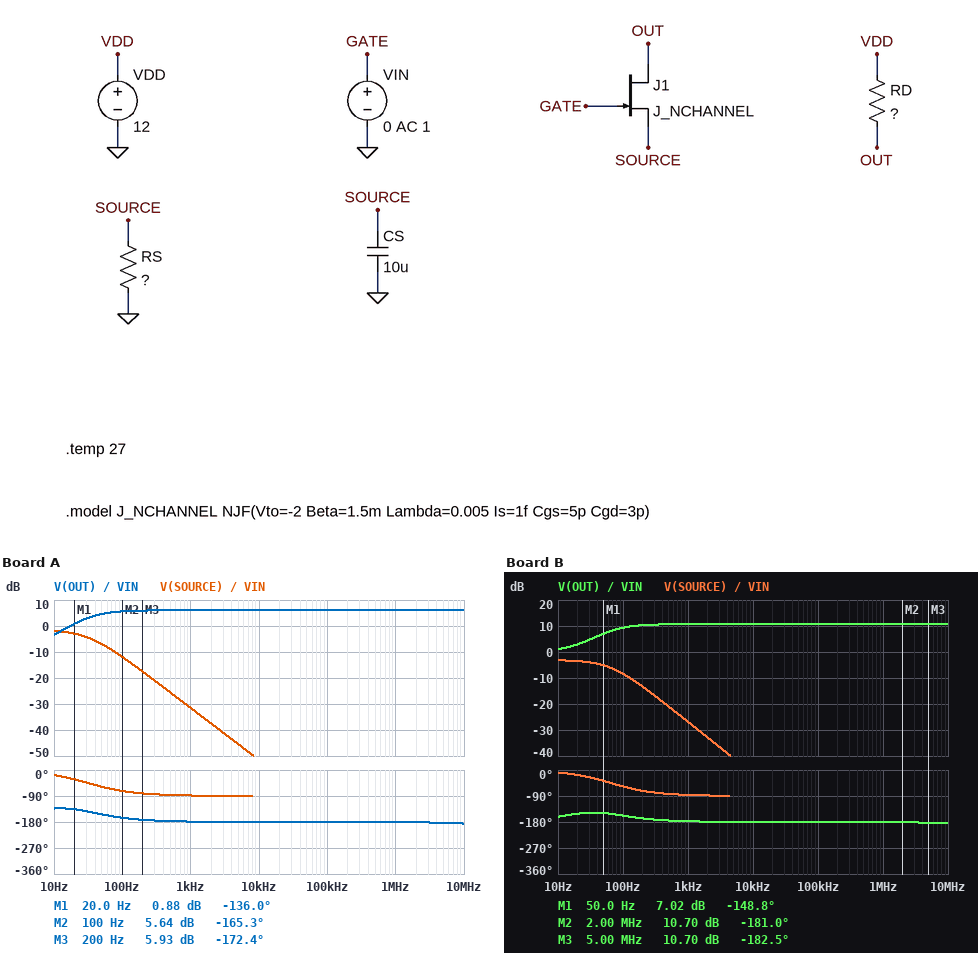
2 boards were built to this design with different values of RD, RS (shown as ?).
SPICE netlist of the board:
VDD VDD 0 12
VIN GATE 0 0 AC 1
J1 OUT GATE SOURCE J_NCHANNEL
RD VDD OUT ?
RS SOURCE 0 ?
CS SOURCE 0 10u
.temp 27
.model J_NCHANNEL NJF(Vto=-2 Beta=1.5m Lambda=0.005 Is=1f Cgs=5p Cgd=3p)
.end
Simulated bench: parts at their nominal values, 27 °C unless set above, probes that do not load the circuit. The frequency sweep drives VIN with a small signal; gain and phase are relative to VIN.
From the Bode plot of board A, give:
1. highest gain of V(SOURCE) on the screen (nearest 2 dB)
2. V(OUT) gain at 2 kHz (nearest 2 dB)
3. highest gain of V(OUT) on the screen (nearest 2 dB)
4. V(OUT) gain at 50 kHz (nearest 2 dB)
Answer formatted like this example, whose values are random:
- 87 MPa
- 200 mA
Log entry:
- -2 dB
- 6 dB
- 6 dB
- 6 dB
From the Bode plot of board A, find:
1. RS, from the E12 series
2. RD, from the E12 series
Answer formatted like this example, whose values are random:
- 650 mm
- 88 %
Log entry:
- 3.3 kΩ
- 1.2 kΩ
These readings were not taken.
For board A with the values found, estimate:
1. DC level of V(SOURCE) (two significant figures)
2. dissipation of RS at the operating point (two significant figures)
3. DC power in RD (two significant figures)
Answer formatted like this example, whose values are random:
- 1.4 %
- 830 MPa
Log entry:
- 1.5 V
- 650 µW
- 240 µW
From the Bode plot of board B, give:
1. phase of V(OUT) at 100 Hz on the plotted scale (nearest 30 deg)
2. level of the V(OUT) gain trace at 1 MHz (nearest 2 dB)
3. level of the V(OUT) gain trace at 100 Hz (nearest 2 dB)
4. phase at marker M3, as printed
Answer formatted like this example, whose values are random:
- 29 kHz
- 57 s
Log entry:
- -150 deg
- 10 dB
- 10 dB
- -182.5 deg
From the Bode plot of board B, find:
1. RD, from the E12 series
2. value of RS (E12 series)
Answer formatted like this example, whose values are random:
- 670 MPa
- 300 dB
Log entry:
- 1.2 kΩ
- 820 Ω
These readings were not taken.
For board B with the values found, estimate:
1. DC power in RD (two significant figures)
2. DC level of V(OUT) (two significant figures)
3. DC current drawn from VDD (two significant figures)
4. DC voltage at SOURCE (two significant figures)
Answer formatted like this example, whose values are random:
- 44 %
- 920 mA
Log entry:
- 2.1 mW
- 10 V
- 1.3 mA
- 1.1 V
